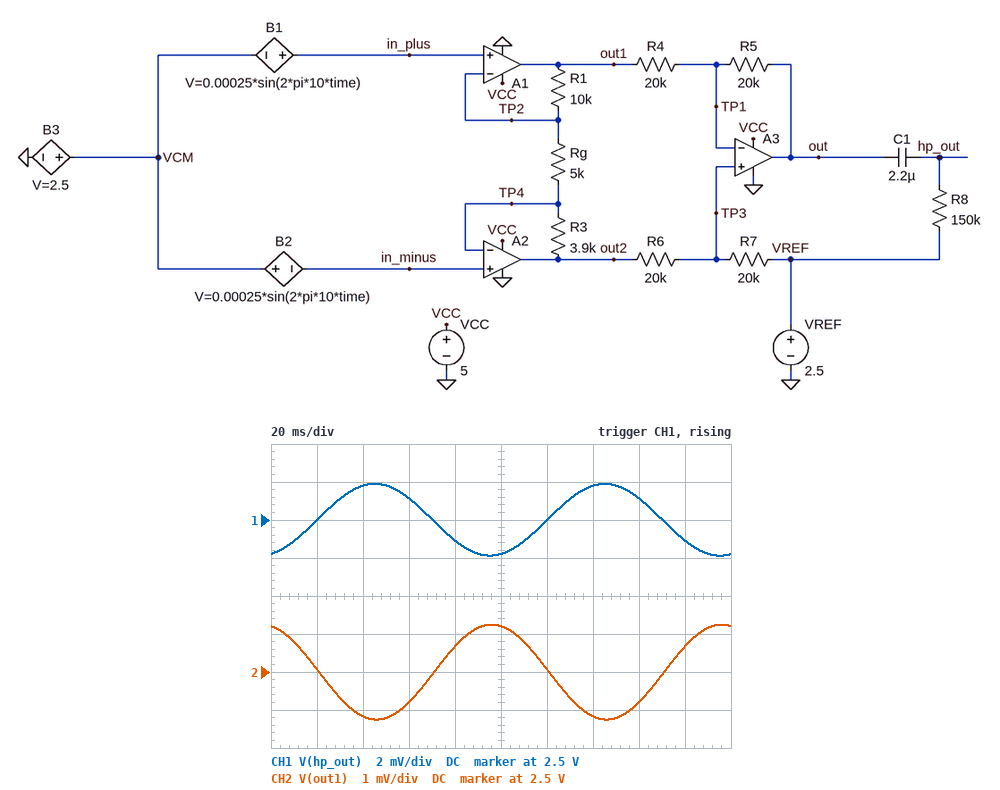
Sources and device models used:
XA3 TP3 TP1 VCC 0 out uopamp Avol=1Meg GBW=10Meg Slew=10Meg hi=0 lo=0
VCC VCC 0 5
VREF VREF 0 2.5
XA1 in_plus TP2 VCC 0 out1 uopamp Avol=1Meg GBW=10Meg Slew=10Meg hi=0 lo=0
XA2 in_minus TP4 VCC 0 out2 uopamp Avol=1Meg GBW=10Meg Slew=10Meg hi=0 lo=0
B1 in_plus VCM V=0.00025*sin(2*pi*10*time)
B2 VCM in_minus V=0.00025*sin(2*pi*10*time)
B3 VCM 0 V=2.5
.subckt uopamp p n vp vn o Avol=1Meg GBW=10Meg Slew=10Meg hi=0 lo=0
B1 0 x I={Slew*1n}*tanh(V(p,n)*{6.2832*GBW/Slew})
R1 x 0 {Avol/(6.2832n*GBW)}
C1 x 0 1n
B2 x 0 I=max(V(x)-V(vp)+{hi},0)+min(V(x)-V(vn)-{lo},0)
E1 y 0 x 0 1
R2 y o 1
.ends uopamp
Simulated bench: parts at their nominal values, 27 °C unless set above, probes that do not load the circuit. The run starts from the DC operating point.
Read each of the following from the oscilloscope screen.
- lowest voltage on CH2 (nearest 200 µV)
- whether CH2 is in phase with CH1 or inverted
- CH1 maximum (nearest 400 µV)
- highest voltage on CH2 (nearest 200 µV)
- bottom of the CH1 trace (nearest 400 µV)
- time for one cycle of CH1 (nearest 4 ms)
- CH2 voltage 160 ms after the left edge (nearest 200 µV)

2.4988 V
inverted
2.5020 V
2.5012 V
2.4980 V
100 ms
2.4992 V
